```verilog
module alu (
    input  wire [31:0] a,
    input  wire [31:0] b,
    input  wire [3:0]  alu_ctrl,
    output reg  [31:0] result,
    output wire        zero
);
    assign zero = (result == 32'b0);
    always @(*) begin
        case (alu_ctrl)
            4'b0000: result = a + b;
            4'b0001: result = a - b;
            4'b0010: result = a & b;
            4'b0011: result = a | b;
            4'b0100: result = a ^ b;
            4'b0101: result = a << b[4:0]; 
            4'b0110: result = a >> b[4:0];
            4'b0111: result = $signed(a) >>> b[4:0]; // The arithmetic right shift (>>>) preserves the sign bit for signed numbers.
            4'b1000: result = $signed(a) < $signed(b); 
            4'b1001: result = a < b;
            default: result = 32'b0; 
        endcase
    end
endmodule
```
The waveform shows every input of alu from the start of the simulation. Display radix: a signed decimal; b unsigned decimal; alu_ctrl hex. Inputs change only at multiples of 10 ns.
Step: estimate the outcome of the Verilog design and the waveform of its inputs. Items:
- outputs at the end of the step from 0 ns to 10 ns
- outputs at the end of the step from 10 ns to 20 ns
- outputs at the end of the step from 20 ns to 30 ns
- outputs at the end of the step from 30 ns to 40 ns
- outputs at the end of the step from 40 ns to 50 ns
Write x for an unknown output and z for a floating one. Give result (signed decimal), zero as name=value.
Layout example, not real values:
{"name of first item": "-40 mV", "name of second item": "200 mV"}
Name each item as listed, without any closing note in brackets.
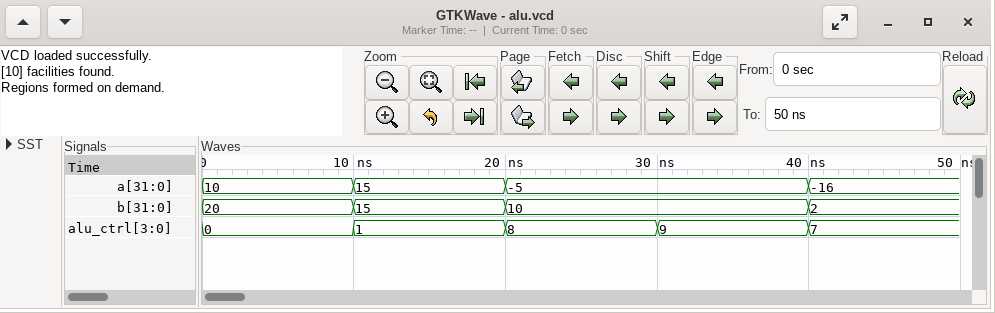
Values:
{"outputs at the end of the step from 0 ns to 10 ns": "result=30, zero=0", "outputs at the end of the step from 10 ns to 20 ns": "result=0, zero=1", "outputs at the end of the step from 20 ns to 30 ns": "result=1, zero=0", "outputs at the end of the step from 30 ns to 40 ns": "result=0, zero=1", "outputs at the end of the step from 40 ns to 50 ns": "result=-4, zero=0"}
